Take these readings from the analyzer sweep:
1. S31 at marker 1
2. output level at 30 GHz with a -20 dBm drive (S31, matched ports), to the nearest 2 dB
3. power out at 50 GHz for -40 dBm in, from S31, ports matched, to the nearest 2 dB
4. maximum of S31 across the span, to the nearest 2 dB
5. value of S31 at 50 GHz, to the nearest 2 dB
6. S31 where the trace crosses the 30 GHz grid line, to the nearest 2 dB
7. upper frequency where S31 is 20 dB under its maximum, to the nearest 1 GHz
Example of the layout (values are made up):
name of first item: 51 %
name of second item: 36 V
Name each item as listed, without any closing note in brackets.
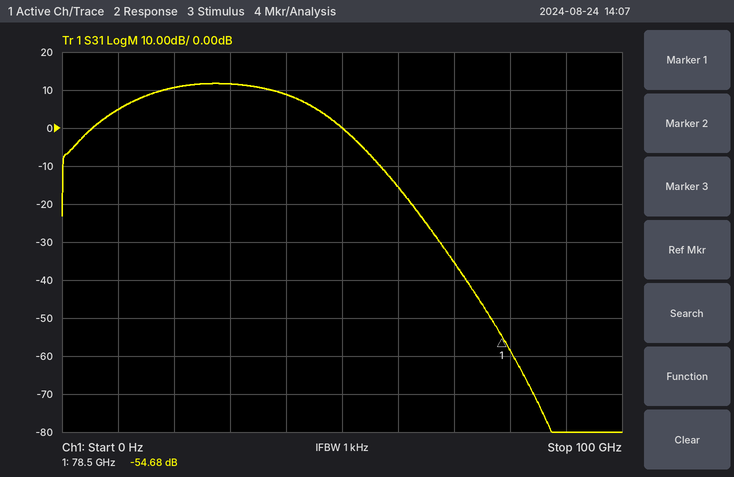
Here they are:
S31 at marker 1: -54.68 dB
output level at 30 GHz with a -20 dBm drive (S31, matched ports), to the nearest 2 dB: -8 dBm
power out at 50 GHz for -40 dBm in, from S31, ports matched, to the nearest 2 dB: -40 dBm
maximum of S31 across the span, to the nearest 2 dB: 12 dB
value of S31 at 50 GHz, to the nearest 2 dB: 0 dB
S31 where the trace crosses the 30 GHz grid line, to the nearest 2 dB: 12 dB
upper frequency where S31 is 20 dB under its maximum, to the nearest 1 GHz: 56 GHz
